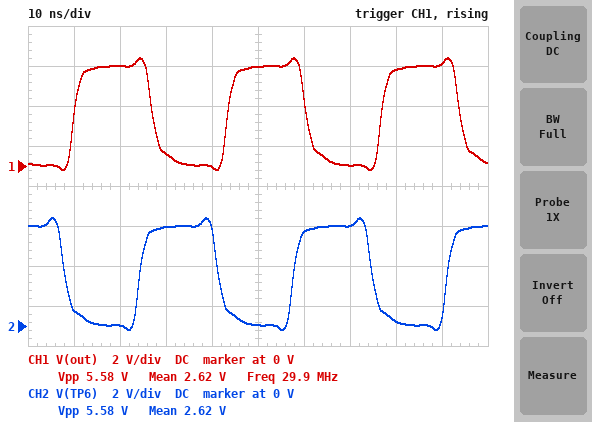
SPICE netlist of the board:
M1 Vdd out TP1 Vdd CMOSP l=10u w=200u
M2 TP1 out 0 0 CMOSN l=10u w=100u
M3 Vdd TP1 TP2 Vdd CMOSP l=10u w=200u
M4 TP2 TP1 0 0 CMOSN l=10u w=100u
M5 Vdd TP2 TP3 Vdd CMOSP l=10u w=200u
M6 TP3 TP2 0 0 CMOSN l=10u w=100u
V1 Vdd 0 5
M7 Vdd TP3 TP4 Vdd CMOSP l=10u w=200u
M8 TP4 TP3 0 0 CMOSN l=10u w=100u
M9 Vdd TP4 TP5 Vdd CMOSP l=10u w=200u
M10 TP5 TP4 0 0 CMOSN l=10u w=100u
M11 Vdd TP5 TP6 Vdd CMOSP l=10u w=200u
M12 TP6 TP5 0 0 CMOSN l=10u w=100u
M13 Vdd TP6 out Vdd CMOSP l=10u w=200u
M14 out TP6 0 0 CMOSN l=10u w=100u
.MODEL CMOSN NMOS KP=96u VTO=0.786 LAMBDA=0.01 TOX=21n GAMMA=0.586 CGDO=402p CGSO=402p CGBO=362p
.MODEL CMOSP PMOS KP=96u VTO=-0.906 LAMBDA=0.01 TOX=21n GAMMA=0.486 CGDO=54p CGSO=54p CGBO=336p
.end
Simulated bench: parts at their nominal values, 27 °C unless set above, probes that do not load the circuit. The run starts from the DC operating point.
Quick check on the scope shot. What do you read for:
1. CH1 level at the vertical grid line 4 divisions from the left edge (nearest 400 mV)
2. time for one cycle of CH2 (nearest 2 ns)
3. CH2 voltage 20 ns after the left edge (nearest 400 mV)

0 V
34 ns
0 V
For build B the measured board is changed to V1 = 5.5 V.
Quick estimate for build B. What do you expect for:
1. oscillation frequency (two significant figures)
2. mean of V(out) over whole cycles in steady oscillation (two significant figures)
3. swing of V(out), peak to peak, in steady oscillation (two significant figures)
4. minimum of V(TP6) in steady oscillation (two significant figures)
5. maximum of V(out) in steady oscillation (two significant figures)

34 MHz
2.9 V
6.1 V
-220 mV
5.9 V
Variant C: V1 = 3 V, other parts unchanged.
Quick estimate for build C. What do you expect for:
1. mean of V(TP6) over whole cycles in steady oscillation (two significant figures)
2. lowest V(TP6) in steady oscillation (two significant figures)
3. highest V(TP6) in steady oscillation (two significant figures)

1.6 V
-160 mV
3.3 V
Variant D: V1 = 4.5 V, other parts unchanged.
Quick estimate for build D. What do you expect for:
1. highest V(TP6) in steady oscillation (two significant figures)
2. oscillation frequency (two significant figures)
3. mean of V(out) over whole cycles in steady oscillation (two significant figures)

4.9 V
26 MHz
2.4 V
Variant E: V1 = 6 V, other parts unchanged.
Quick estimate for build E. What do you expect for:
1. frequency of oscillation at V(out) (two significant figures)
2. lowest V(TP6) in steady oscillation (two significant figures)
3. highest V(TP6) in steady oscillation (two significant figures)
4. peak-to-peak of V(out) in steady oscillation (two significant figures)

39 MHz
-230 mV
6.4 V
6.7 V
